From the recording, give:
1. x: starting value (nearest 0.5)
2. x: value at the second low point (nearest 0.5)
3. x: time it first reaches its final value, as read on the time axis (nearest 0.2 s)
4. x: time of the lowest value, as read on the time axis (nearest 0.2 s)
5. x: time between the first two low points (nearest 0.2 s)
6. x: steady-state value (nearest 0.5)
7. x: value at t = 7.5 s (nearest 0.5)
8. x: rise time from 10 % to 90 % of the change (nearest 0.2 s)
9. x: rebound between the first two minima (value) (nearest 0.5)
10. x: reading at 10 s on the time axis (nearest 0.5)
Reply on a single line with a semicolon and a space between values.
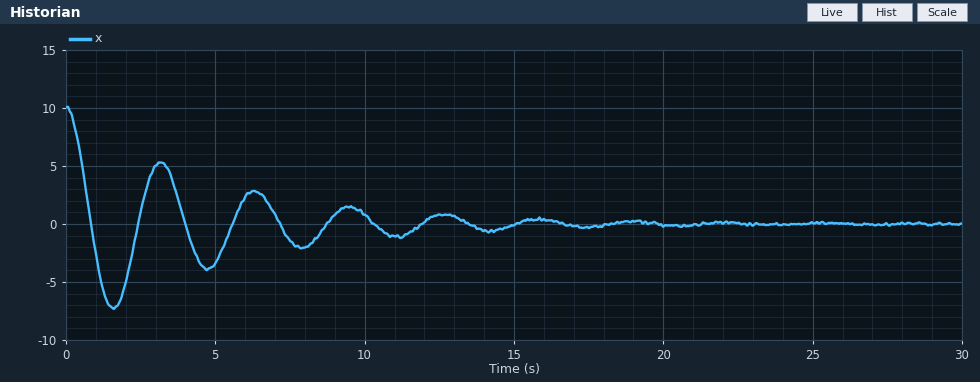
10.0; -4.0; 0.8 s; 1.6 s; 3.2 s; 0.0; -1.5; 0.6 s; 5.5; 1.0
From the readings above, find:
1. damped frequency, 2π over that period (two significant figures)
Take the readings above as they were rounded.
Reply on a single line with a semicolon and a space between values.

2.0 rad/s
